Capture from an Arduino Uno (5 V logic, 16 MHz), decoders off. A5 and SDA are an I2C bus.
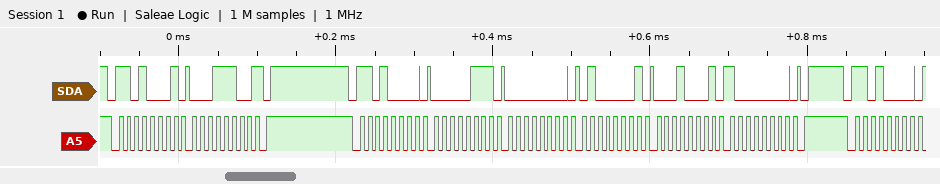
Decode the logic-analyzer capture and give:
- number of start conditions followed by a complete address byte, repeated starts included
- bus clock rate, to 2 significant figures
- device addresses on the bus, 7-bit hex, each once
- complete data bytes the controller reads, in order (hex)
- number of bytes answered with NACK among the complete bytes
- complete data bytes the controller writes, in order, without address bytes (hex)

3
100 kHz
0x68
1C
1
07 00 41 11 80
